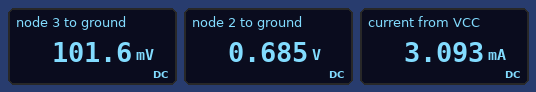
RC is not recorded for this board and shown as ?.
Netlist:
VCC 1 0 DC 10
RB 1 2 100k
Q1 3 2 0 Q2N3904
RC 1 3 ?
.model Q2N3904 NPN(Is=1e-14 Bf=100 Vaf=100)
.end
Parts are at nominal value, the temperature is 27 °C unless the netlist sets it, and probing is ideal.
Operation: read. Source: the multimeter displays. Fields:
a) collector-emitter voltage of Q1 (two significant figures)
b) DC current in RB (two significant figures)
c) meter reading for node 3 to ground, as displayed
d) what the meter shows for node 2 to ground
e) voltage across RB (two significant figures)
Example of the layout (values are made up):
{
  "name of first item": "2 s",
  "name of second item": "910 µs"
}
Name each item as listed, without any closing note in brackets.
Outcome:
{
  "collector-emitter voltage of Q1": "100 mV",
  "DC current in RB": "93 µA",
  "meter reading for node 3 to ground, as displayed": "101.6 mV",
  "what the meter shows for node 2 to ground": "0.685 V",
  "voltage across RB": "9.3 V"
}
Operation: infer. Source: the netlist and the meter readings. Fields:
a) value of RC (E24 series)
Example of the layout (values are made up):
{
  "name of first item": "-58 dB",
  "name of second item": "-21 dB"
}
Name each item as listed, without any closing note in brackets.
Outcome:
{
  "value of RC": "3.3 kΩ"
}
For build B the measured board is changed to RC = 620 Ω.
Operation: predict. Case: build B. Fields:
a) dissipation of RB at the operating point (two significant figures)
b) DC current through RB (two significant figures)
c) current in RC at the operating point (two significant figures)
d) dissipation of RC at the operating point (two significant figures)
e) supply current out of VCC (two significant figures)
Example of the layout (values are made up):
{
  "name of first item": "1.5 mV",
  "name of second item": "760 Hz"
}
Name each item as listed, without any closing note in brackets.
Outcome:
{
  "dissipation of RB at the operating point": "860 µW",
  "DC current through RB": "93 µA",
  "current in RC at the operating point": "9.6 mA",
  "dissipation of RC at the operating point": "57 mW",
  "supply current out of VCC": "9.7 mA"
}
